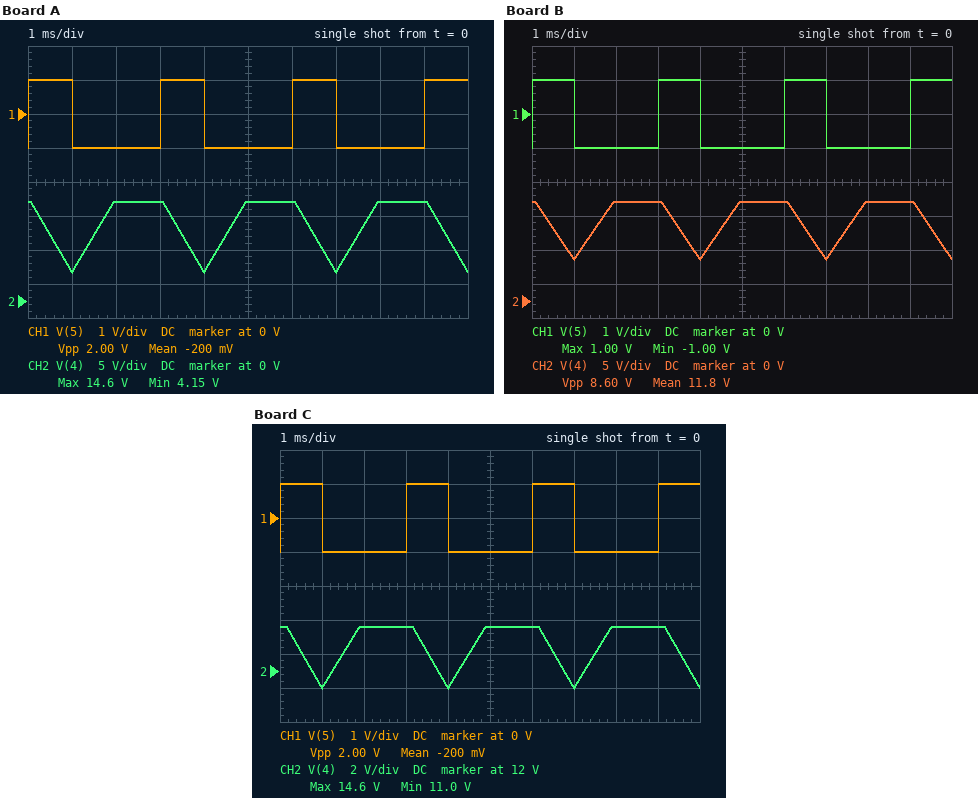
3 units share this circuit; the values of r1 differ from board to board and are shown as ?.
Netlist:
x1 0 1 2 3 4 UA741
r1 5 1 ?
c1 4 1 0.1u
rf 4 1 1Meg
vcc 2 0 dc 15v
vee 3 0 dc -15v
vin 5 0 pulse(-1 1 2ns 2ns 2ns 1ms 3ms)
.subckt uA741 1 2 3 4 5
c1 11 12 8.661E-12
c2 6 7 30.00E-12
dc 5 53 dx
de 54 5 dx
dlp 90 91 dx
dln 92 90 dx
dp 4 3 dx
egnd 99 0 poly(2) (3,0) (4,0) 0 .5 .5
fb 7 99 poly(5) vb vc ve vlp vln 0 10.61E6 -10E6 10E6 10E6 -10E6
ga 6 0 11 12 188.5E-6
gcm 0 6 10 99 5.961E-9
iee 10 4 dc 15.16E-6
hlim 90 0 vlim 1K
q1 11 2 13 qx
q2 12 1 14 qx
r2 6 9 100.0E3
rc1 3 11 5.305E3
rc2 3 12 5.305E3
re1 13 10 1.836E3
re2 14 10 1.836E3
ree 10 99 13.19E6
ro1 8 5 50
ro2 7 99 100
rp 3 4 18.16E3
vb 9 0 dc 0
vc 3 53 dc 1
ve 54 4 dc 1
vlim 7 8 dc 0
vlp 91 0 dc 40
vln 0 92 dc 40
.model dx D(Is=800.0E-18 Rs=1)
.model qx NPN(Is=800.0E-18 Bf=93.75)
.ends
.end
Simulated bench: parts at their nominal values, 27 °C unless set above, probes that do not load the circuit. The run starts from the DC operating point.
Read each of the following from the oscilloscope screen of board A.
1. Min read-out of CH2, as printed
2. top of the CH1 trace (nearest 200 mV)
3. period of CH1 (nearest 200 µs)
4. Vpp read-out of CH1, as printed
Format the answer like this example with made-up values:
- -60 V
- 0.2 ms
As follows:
- 4.15 V
- 1.0 V
- 3.0 ms
- 2.00 V
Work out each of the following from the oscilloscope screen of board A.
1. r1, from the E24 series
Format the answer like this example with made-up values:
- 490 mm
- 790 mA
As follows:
- 910 Ω
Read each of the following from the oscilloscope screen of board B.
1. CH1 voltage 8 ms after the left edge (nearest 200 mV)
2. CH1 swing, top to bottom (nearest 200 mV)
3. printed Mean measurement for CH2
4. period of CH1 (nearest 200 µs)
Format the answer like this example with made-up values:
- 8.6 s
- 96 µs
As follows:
- -1.0 V
- 2.0 V
- 11.8 V
- 3.0 ms
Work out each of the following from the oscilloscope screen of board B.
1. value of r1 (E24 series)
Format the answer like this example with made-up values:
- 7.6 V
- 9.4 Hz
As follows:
- 1.1 kΩ
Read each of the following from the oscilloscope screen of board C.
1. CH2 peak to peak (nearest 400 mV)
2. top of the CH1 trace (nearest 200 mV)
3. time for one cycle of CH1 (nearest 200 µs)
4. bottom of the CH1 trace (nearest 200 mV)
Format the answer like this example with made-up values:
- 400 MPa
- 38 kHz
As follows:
- 3.6 V
- 1.0 V
- 3.0 ms
- -1.0 V
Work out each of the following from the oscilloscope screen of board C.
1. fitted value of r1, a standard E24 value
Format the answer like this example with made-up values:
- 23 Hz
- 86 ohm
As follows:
- 2.4 kΩ
